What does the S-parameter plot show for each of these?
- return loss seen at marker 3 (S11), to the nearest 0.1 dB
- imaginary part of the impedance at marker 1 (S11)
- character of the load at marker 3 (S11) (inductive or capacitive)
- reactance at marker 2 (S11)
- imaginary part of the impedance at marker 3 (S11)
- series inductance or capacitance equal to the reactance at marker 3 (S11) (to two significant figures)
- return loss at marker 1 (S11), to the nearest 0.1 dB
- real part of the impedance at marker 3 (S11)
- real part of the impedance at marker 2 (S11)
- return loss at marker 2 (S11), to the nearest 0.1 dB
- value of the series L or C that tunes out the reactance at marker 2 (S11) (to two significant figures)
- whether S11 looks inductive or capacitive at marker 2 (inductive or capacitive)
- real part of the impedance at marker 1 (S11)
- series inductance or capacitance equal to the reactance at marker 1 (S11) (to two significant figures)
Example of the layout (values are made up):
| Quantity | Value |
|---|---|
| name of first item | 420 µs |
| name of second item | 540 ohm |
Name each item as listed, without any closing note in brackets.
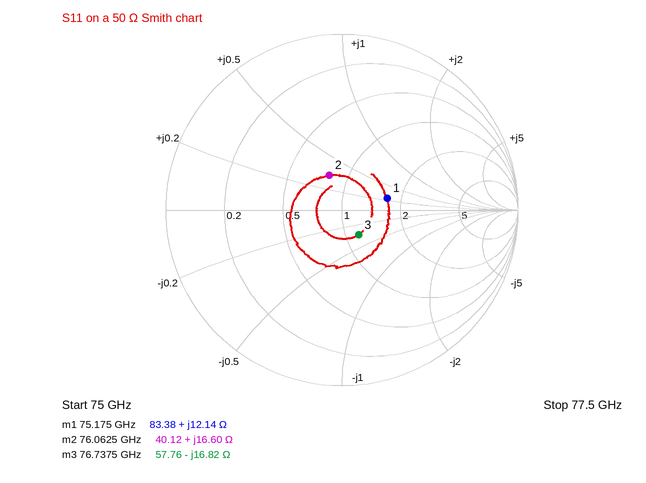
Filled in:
| Quantity | Value |
|---|---|
| return loss seen at marker 3 (S11), to the nearest 0.1 dB | 15.4 dB |
| imaginary part of the impedance at marker 1 | +12.14 Ω |
| character of the load at marker 3 (S11) | capacitive |
| reactance at marker 2 | +16.60 Ω |
| imaginary part of the impedance at marker 3 | -16.82 Ω |
| series inductance or capacitance equal to the reactance at marker 3 (S11) | 120 fF |
| return loss at marker 1 (S11), to the nearest 0.1 dB | 11.5 dB |
| real part of the impedance at marker 3 | 57.76 Ω |
| real part of the impedance at marker 2 | 40.12 Ω |
| return loss at marker 2 (S11), to the nearest 0.1 dB | 13.5 dB |
| value of the series L or C that tunes out the reactance at marker 2 (S11) | 130 fF |
| whether S11 looks inductive or capacitive at marker 2 | inductive |
| real part of the impedance at marker 1 | 83.38 Ω |
| series inductance or capacitance equal to the reactance at marker 1 (S11) | 26 pH |
